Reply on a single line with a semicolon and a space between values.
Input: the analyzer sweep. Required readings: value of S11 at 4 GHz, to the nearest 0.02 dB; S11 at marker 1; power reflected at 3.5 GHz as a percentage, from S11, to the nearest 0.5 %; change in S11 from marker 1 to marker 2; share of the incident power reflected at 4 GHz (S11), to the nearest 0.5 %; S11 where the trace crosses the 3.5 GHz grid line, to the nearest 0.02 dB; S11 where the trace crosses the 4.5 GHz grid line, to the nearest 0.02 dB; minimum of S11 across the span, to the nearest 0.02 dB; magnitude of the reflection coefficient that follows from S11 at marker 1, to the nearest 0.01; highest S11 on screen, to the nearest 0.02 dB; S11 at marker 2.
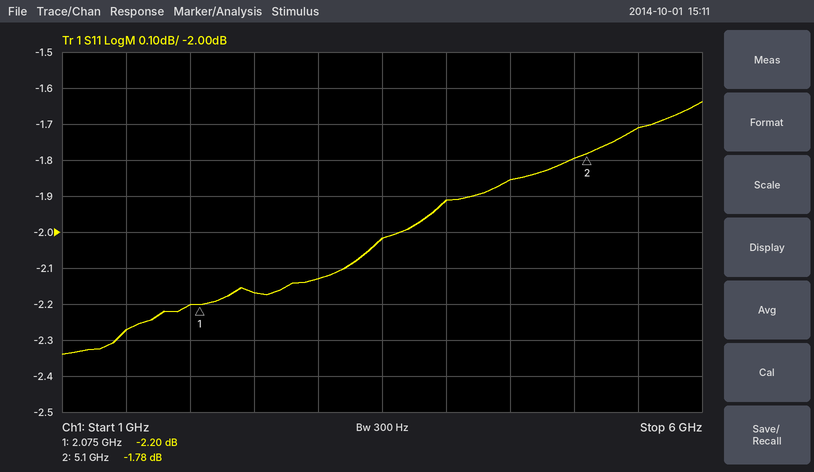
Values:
-1.92 dB; -2.20 dB; 63.0 %; 0.42 dB; 64.5 %; -2.02 dB; -1.86 dB; -2.34 dB; 0.78; -1.64 dB; -1.78 dB
